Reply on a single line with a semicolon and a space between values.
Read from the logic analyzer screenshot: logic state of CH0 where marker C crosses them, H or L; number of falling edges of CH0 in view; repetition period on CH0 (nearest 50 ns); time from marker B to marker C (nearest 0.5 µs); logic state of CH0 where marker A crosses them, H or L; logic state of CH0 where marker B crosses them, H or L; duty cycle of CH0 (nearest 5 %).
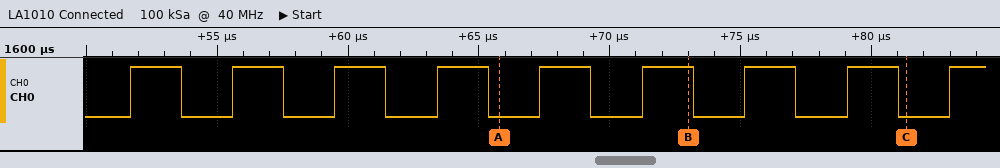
CH0=L; 8; 3900 ns; 8.5 µs; CH0=L; CH0=H; 50 %
